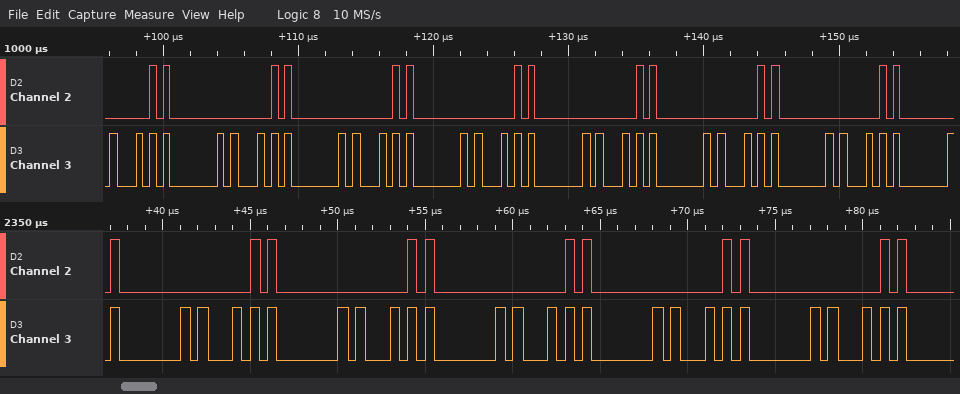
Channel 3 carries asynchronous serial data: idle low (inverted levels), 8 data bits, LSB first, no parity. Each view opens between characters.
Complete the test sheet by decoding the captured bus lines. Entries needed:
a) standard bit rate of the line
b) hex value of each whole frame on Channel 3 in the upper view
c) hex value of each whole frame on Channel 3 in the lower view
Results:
2000000 baud
57, 5D, 7F, 57, 5D, 7F, 57, 5D, 7F, 57
7F, 57, 5D, 7F, 57, 5D, 7F, 57
